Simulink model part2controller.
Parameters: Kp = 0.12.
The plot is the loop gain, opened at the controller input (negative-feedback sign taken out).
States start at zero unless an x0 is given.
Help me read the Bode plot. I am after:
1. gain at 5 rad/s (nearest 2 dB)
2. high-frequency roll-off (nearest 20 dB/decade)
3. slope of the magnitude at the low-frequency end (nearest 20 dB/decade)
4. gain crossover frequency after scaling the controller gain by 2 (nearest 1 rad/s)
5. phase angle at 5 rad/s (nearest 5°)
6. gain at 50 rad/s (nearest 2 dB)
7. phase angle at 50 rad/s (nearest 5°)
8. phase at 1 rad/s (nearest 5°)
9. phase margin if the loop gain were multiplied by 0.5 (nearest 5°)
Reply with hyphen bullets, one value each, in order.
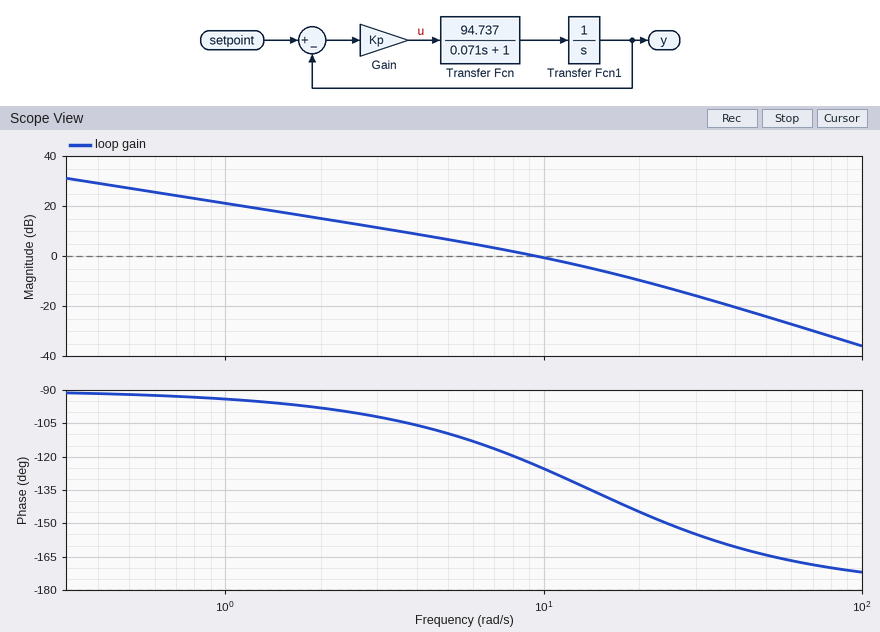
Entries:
- 6 dB
- -40 dB/decade
- -20 dB/decade
- 15 rad/s
- -110°
- -24 dB
- -165°
- -95°
- 70°
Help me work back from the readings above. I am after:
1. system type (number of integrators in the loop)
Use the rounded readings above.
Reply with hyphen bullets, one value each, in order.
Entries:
- 1
